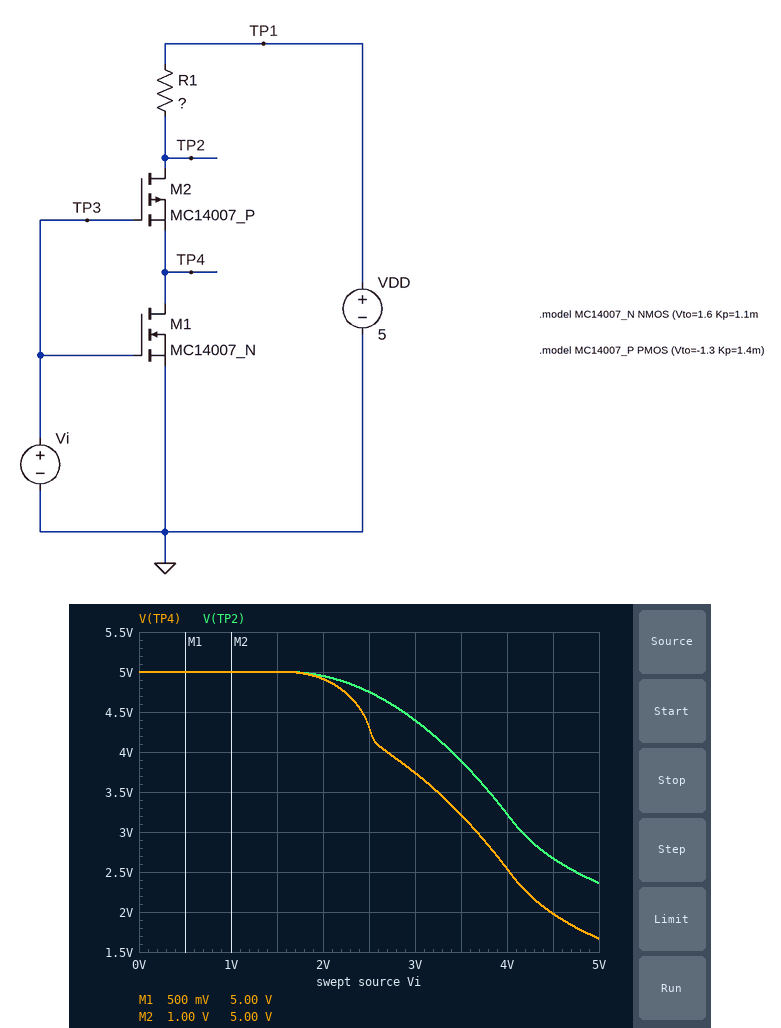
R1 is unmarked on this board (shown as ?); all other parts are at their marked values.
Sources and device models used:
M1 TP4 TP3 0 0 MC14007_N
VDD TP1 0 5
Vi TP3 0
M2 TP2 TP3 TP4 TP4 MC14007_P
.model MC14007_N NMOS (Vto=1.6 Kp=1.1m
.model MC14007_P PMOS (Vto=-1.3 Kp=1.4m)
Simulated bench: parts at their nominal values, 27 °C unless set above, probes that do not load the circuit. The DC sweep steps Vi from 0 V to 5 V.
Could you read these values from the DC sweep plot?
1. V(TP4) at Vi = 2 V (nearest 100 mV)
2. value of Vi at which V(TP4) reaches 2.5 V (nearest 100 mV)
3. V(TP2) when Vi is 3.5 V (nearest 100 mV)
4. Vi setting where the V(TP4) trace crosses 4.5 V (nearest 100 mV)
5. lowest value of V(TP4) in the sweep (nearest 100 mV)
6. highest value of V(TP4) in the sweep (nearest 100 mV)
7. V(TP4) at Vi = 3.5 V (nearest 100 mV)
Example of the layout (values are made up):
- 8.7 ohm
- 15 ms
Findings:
- 4.9 V
- 4.0 V
- 3.9 V
- 2.4 V
- 1.7 V
- 5.0 V
- 3.2 V
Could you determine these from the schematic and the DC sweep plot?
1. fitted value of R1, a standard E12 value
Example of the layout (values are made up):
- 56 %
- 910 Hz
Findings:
- 560 Ω
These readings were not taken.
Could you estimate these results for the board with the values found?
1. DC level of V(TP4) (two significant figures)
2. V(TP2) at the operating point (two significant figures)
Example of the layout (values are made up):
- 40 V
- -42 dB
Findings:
- 5.0 V
- 5.0 V
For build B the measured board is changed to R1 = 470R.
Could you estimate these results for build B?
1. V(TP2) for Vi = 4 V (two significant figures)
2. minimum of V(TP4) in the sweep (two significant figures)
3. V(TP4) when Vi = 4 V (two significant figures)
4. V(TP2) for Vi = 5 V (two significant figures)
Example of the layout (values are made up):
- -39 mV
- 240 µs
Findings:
- 3.5 V
- 1.9 V
- 2.8 V
- 2.6 V
